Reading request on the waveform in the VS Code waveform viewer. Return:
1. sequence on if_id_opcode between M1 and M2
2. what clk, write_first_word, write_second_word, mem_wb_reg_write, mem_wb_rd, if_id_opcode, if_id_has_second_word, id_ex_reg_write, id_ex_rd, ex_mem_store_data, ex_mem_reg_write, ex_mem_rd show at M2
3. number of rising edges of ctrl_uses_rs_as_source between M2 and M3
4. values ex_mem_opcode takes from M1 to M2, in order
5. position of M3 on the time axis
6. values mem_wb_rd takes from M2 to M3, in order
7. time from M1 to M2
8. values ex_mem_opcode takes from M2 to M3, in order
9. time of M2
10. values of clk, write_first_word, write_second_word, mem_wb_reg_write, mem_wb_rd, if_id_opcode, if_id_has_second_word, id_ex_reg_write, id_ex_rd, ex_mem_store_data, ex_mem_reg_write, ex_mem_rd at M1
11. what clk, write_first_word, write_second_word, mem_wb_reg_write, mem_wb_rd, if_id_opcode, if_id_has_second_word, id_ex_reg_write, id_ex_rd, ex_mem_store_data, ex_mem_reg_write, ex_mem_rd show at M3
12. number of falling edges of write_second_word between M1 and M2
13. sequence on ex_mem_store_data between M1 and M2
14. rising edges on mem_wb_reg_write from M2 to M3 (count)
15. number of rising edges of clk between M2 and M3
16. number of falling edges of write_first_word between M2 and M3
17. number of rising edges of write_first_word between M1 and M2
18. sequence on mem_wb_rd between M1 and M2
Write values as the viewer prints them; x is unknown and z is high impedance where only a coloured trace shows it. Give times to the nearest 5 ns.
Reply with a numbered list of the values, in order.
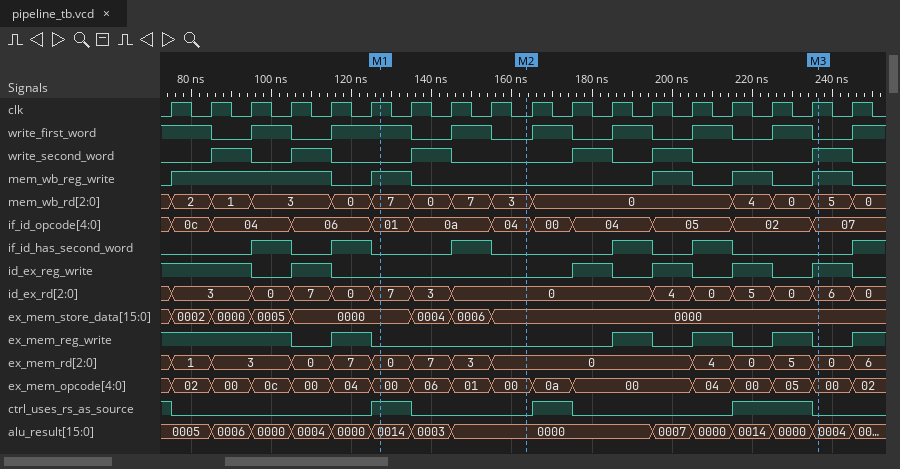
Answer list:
1. 01, 0a, 04
2. clk=0, write_first_word=0, write_second_word=0, mem_wb_reg_write=0, mem_wb_rd=3, if_id_opcode=04, if_id_has_second_word=0, id_ex_reg_write=0, id_ex_rd=0, ex_mem_store_data=0000, ex_mem_reg_write=0, ex_mem_rd=0
3. 2
4. 00, 06, 01, 00
5. 235 ns
6. 3, 0, 4, 0, 5
7. 35 ns
8. 00, 0a, 00, 04, 00, 05, 00
9. 165 ns
10. clk=1, write_first_word=1, write_second_word=0, mem_wb_reg_write=1, mem_wb_rd=7, if_id_opcode=01, if_id_has_second_word=0, id_ex_reg_write=0, id_ex_rd=7, ex_mem_store_data=0000, ex_mem_reg_write=0, ex_mem_rd=0
11. clk=1, write_first_word=0, write_second_word=1, mem_wb_reg_write=1, mem_wb_rd=5, if_id_opcode=07, if_id_has_second_word=0, id_ex_reg_write=1, id_ex_rd=6, ex_mem_store_data=0000, ex_mem_reg_write=0, ex_mem_rd=0
12. 1
13. 0000, 0004, 0006, 0000
14. 3
15. 8
16. 4
17. 1
18. 7, 0, 7, 3
